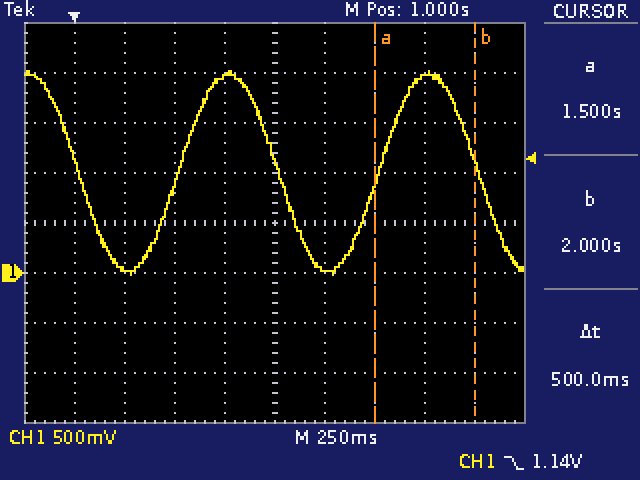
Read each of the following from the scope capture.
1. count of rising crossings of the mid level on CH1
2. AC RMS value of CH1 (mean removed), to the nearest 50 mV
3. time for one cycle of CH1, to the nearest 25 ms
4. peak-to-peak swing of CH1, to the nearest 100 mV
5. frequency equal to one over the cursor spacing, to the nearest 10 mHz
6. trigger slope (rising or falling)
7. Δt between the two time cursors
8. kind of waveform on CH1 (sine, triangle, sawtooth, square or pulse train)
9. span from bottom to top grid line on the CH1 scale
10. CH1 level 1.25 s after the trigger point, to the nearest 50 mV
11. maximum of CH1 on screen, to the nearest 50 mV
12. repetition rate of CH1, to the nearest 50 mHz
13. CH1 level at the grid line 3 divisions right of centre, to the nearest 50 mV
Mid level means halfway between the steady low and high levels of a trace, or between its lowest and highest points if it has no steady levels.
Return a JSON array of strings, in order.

["2", "700 mV", "1.000 s", "2.00 V", "2.00 Hz", "falling", "500 ms", "sine", "4 V", "50 mV", "2.00 V", "1.00 Hz", "1.95 V"]
